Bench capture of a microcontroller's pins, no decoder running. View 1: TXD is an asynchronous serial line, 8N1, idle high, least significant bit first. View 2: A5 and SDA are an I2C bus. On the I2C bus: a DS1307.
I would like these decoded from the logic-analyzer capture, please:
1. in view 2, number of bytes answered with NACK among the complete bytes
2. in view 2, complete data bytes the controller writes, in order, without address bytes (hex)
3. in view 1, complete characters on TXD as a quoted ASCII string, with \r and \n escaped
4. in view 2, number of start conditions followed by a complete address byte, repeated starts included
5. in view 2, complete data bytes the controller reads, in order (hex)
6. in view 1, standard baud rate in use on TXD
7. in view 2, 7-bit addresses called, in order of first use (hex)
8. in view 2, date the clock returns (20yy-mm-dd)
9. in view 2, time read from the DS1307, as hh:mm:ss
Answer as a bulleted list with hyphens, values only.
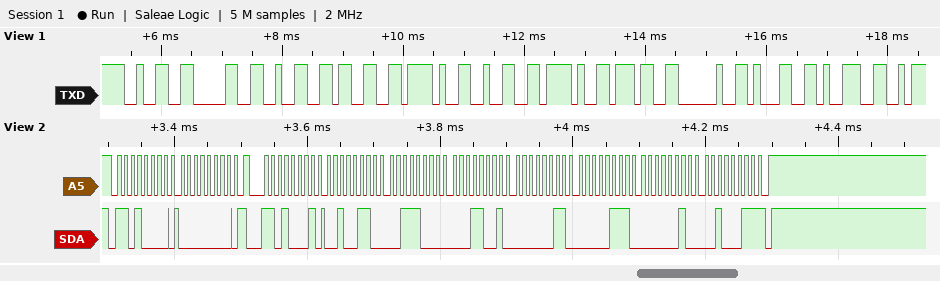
- 1
- 00
- "2023/2/7 19"
- 2
- 26 38 19 03 07 02 23
- 9600 baud
- 0x68
- 2023-02-07
- 19:38:26
